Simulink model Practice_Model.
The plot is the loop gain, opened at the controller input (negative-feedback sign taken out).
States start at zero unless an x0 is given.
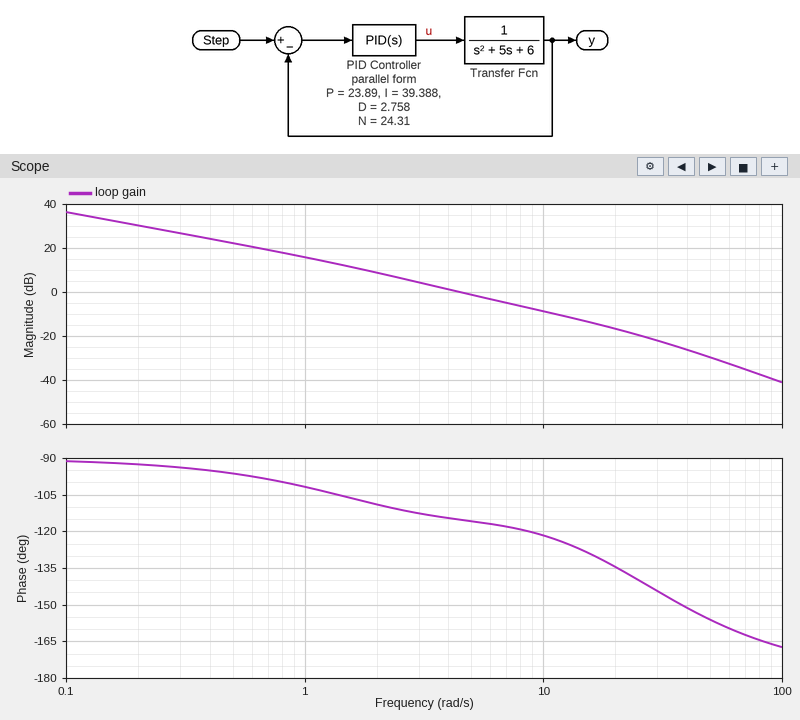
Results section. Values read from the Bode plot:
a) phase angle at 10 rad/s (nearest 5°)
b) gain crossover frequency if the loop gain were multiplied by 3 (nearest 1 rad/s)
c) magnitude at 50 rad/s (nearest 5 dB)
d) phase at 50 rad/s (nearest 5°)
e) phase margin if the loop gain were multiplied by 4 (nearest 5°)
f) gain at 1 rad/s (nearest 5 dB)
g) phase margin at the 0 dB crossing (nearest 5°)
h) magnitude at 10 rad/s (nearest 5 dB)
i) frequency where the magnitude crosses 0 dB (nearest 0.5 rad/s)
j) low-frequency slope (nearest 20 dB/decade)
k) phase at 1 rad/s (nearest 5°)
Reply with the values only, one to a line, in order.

-120°
11 rad/s
-30 dB
-155°
55°
15 dB
65°
-10 dB
4.5 rad/s
-20 dB/decade
-100°
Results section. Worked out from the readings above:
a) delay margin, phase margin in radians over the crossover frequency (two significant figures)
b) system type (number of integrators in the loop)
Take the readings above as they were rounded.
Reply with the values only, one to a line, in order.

0.25 s
1
